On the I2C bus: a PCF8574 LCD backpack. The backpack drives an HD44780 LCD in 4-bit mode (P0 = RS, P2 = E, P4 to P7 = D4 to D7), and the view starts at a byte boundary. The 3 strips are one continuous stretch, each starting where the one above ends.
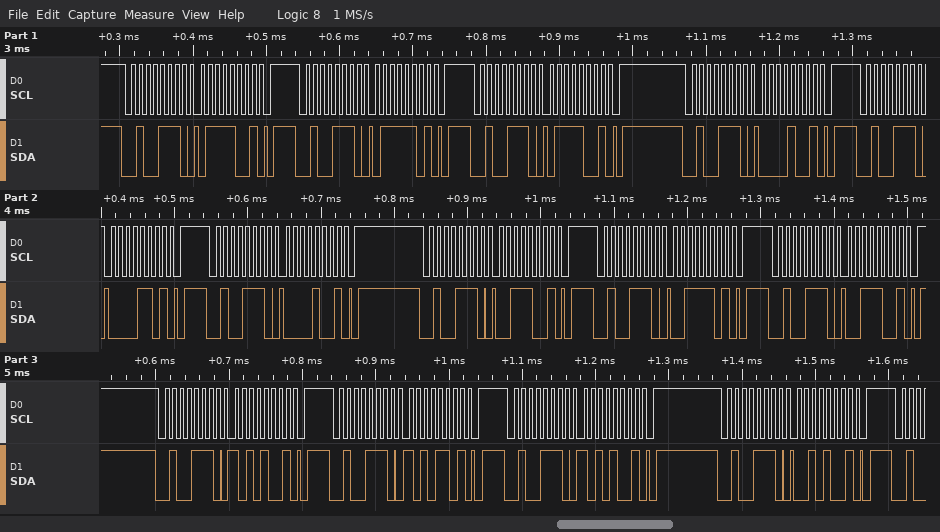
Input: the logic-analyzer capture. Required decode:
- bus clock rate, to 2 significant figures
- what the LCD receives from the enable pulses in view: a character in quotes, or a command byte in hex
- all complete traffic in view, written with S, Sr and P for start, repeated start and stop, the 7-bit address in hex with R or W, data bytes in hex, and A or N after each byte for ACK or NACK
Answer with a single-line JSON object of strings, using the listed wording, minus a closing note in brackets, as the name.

{"bus clock rate, to 2 significant figures": "100 kHz", "what the LCD receives from the enable pulses in view: a character in quotes, or a command byte in hex": "'p' ':'", "all complete traffic in view, written with S, Sr and P for start, repeated start and stop, the 7-bit address in hex with R or W, data bytes in hex, and A or N after each byte for ACK or NACK": "S 27W A 79 A P S 27W A 7D A P S 27W A 79 A P S 27W A 09 A P S 27W A 0D A P S 27W A 09 A P S 27W A 39 A P S 27W A 3D A P S 27W A 39 A P S 27W A A9 A P S 27W A AD A P S 27W A A9 A P S 27W A 29 A P"}
